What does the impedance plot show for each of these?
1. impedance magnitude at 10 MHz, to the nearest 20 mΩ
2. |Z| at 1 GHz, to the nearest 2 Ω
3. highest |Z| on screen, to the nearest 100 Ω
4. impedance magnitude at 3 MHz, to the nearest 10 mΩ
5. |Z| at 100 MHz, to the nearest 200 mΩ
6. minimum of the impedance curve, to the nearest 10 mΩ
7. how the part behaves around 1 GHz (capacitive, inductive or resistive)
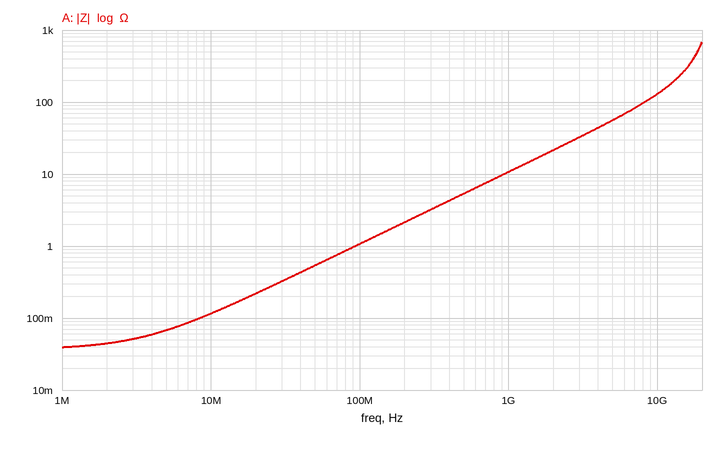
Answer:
120 mΩ
10 Ω
700 Ω
50 mΩ
1.0 Ω
40 mΩ
inductive
